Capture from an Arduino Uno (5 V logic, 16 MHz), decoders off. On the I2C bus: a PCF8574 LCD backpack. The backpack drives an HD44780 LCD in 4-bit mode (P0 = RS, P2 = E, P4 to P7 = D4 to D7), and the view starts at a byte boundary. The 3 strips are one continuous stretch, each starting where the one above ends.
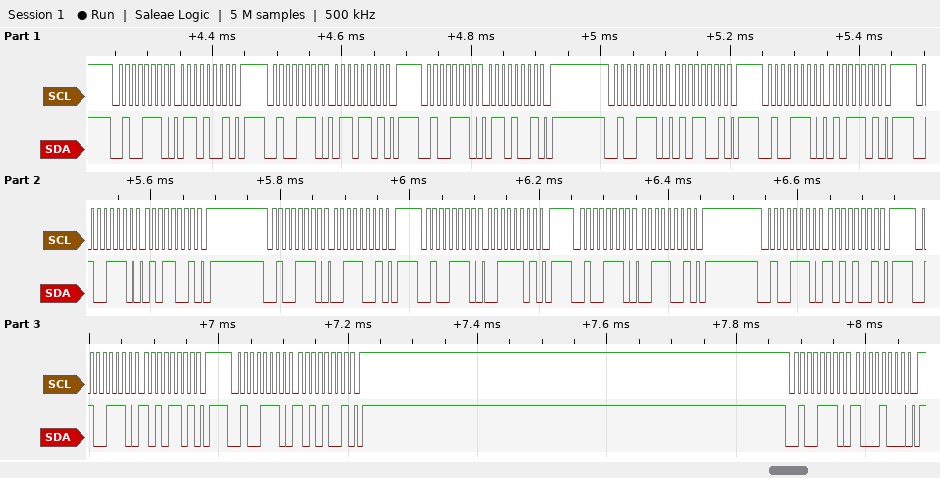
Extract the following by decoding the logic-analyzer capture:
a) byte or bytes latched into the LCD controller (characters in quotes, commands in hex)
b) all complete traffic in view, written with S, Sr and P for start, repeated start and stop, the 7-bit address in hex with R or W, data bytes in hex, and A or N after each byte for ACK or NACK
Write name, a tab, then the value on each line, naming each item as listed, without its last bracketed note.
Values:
byte or bytes latched into the LCD controller	'e' ':'
all complete traffic in view, written with S, Sr and P for start, repeated start and stop, the 7-bit address in hex with R or W, data bytes in hex, and A or N after each byte for ACK or NACK	S 27W A 69 A P S 27W A 6D A P S 27W A 69 A P S 27W A 59 A P S 27W A 5D A P S 27W A 59 A P S 27W A 39 A P S 27W A 3D A P S 27W A 39 A P S 27W A A9 A P S 27W A AD A P S 27W A A9 A P S 27W A 88 A P
